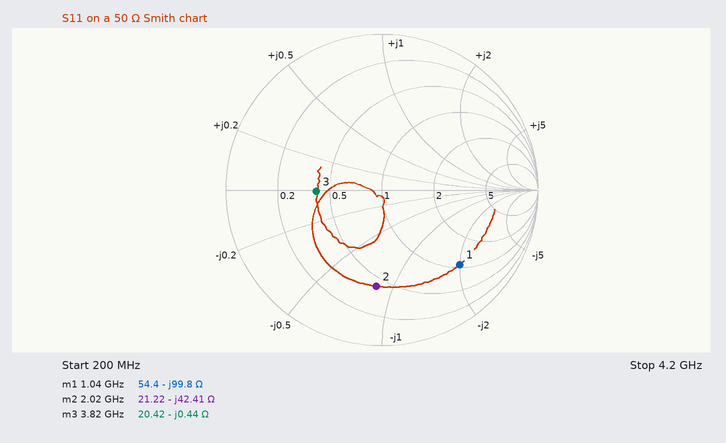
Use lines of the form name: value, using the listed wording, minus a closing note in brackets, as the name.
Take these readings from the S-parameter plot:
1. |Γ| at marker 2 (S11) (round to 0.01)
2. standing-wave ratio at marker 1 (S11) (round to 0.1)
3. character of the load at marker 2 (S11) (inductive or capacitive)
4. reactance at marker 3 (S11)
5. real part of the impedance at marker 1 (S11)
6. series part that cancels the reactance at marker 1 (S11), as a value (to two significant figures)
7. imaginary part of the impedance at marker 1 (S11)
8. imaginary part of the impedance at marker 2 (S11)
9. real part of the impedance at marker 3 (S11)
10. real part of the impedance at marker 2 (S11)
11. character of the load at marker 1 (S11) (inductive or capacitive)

|Γ| at marker 2 (S11): 0.62
standing-wave ratio at marker 1 (S11): 5.5
character of the load at marker 2 (S11): capacitive
reactance at marker 3: -0.44 Ω
real part of the impedance at marker 1: 54.4 Ω
series part that cancels the reactance at marker 1 (S11), as a value: 15 nH
imaginary part of the impedance at marker 1: -99.8 Ω
imaginary part of the impedance at marker 2: -42.41 Ω
real part of the impedance at marker 3: 20.42 Ω
real part of the impedance at marker 2: 21.22 Ω
character of the load at marker 1 (S11): capacitive
